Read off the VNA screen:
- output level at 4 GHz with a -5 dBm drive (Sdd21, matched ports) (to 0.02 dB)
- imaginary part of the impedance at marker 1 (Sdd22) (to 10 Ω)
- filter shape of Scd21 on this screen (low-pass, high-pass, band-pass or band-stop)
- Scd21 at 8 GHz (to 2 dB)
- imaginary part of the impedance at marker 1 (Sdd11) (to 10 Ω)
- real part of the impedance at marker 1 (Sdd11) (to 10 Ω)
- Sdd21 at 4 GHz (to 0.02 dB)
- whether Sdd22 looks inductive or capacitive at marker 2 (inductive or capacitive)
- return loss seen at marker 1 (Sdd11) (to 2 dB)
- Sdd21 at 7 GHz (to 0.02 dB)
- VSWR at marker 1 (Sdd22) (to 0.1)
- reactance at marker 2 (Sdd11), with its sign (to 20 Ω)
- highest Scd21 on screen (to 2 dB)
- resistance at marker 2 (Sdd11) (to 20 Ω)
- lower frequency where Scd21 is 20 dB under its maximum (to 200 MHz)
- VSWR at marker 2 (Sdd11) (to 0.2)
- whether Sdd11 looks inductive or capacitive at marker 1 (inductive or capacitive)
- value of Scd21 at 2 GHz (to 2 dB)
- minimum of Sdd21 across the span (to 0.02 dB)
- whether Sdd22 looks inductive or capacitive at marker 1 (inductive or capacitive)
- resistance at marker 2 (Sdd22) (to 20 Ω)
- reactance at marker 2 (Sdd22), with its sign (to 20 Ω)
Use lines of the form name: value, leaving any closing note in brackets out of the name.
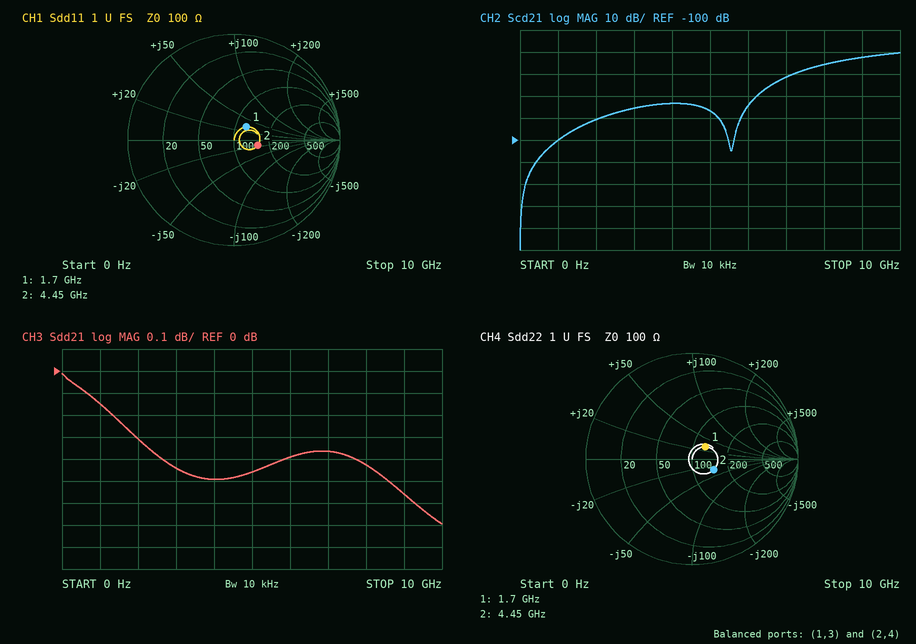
output level at 4 GHz with a -5 dBm drive (Sdd21, matched ports): -5.50 dBm
imaginary part of the impedance at marker 1 (Sdd22): +30 Ω
filter shape of Scd21 on this screen: high-pass
Scd21 at 8 GHz: -66 dB
imaginary part of the impedance at marker 1 (Sdd11): +30 Ω
real part of the impedance at marker 1 (Sdd11): 120 Ω
Sdd21 at 4 GHz: -0.50 dB
whether Sdd22 looks inductive or capacitive at marker 2: capacitive
return loss seen at marker 1 (Sdd11): 16 dB
Sdd21 at 7 GHz: -0.36 dB
VSWR at marker 1 (Sdd22): 1.4
reactance at marker 2 (Sdd11), with its sign: -20 Ω
highest Scd21 on screen: -60 dB
resistance at marker 2 (Sdd11): 160 Ω
lower frequency where Scd21 is 20 dB under its maximum: 6.2 GHz
VSWR at marker 2 (Sdd11): 1.6
whether Sdd11 looks inductive or capacitive at marker 1: inductive
value of Scd21 at 2 GHz: -90 dB
minimum of Sdd21 across the span: -0.70 dB
whether Sdd22 looks inductive or capacitive at marker 1: inductive
resistance at marker 2 (Sdd22): 140 Ω
reactance at marker 2 (Sdd22), with its sign: -40 Ω
